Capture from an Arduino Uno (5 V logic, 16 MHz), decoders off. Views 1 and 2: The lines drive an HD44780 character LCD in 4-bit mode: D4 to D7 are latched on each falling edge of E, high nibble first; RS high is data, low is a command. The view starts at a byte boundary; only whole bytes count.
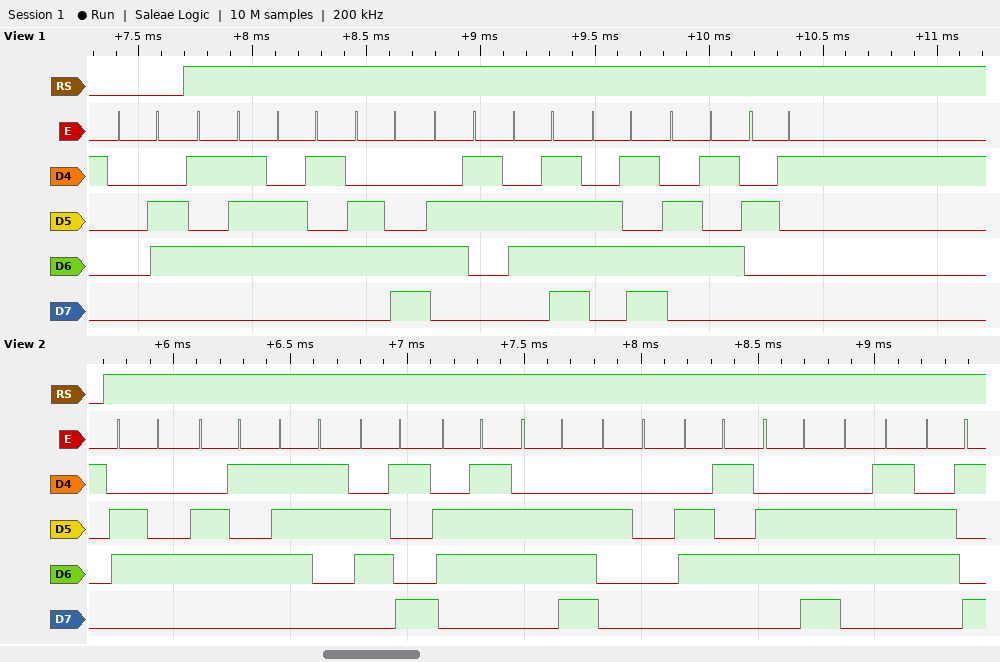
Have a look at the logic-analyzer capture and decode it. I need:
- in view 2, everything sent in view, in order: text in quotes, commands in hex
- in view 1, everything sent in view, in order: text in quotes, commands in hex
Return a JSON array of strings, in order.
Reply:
["\"design engi\"", "0x06 \"Welcome!\""]
